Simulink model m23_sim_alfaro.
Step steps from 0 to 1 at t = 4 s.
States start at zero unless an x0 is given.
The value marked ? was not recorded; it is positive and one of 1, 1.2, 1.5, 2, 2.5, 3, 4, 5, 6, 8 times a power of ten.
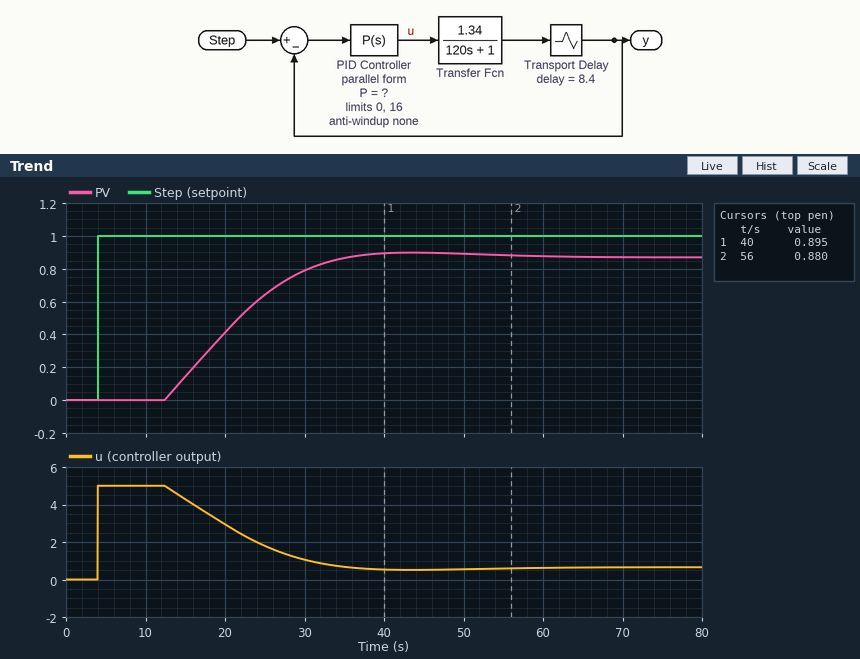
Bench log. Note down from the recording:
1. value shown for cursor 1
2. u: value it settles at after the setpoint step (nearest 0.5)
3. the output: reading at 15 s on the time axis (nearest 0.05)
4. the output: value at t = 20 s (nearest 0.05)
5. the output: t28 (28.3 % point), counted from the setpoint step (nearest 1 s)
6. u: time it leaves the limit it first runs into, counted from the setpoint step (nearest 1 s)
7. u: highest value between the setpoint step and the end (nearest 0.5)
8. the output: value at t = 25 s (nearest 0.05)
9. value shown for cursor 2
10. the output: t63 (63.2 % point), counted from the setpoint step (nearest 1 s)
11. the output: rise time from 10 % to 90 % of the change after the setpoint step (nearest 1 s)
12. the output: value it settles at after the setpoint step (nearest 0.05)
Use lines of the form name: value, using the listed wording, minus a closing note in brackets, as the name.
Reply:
value shown for cursor 1: 0.895
u: value it settles at after the setpoint step: 0.5
the output: reading at 15 s on the time axis: 0.15
the output: value at t = 20 s: 0.40
the output: t28 (28.3 % point), counted from the setpoint step: 13 s
u: time it leaves the limit it first runs into, counted from the setpoint step: 9 s
u: highest value between the setpoint step and the end: 5.0
the output: value at t = 25 s: 0.65
value shown for cursor 2: 0.880
the output: t63 (63.2 % point), counted from the setpoint step: 19 s
the output: rise time from 10 % to 90 % of the change after the setpoint step: 16 s
the output: value it settles at after the setpoint step: 0.85
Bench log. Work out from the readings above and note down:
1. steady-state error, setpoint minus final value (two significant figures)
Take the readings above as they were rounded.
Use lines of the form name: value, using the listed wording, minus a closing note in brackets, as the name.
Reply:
steady-state error, setpoint minus final value: 0.15
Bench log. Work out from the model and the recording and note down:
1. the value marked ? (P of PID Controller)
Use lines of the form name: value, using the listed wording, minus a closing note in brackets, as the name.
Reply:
the value marked ?: 5
